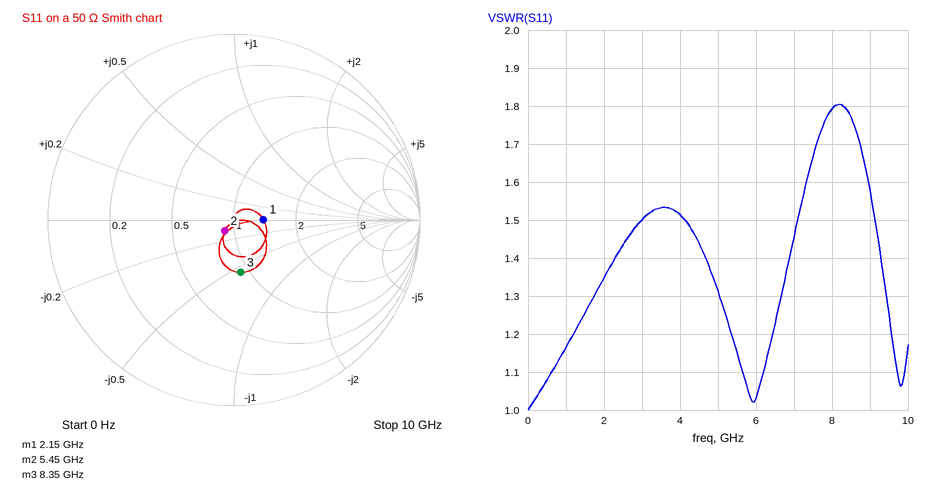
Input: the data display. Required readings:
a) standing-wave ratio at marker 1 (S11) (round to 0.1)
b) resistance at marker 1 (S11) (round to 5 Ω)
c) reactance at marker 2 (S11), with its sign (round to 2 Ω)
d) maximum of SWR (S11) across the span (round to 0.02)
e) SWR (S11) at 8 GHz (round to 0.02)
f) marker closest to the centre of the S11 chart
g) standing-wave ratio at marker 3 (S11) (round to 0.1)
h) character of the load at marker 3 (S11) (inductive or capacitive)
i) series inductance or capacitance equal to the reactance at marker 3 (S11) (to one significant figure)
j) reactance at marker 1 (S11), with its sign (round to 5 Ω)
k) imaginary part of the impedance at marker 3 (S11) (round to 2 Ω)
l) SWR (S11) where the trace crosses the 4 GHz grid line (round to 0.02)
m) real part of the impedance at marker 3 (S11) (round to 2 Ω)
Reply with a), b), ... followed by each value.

a) 1.4
b) 70 Ω
c) -6 Ω
d) 1.80
e) 1.80
f) marker 2
g) 1.8
h) capacitive
i) 700 fF
j) 0 Ω
k) -28 Ω
l) 1.52
m) 46 Ω
